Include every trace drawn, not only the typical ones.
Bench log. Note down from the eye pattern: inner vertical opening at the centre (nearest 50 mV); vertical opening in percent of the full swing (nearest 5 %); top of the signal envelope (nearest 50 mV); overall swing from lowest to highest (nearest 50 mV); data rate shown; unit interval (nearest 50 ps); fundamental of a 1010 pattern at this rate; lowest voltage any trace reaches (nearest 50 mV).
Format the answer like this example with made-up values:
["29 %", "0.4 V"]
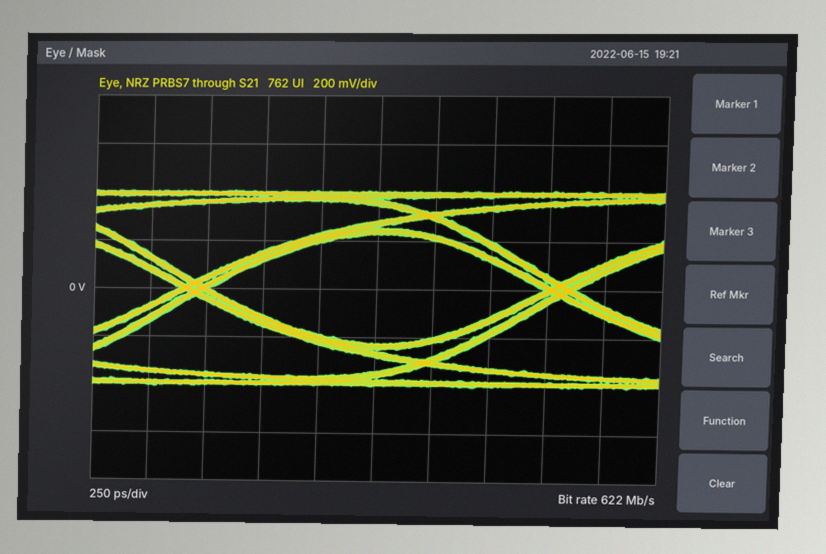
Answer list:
["450 mV", "55 %", "400 mV", "800 mV", "622 Mb/s", "1.60 ns", "311 MHz", "-400 mV"]
